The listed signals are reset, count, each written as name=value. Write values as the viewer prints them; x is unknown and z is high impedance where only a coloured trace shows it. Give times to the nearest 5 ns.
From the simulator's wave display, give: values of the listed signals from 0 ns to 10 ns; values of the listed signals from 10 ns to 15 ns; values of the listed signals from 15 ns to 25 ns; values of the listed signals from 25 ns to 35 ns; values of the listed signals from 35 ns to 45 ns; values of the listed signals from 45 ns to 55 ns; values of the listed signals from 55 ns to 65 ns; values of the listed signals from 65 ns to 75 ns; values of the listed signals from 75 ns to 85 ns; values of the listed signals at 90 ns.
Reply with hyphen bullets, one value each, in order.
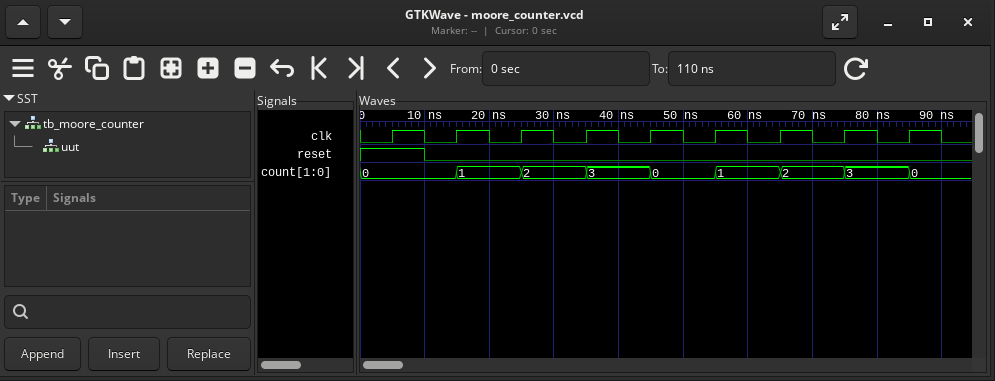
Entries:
- reset=1, count=0
- reset=0, count=0
- reset=0, count=1
- reset=0, count=2
- reset=0, count=3
- reset=0, count=0
- reset=0, count=1
- reset=0, count=2
- reset=0, count=3
- reset=0, count=0
